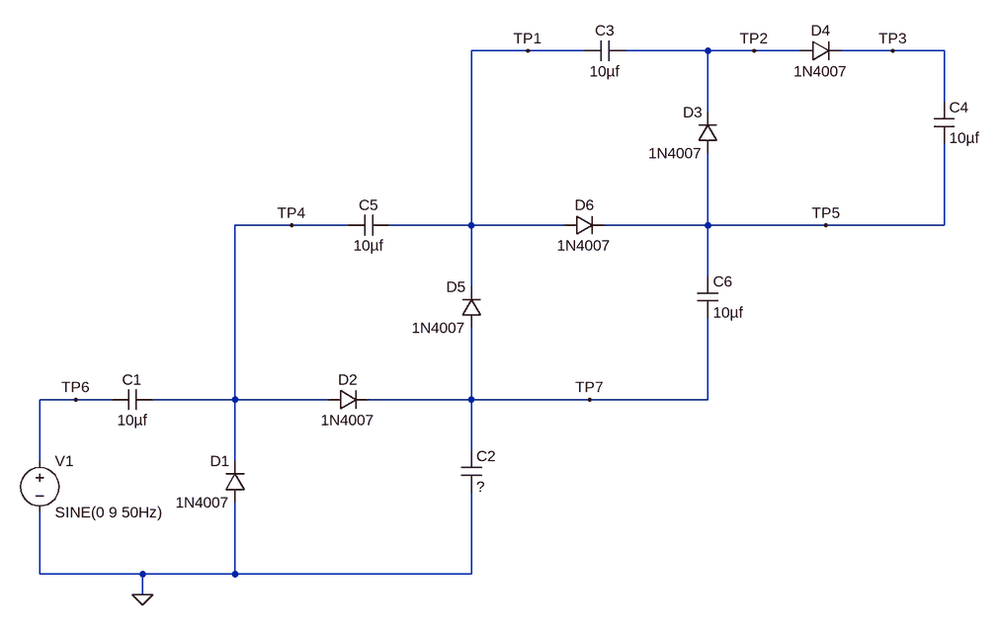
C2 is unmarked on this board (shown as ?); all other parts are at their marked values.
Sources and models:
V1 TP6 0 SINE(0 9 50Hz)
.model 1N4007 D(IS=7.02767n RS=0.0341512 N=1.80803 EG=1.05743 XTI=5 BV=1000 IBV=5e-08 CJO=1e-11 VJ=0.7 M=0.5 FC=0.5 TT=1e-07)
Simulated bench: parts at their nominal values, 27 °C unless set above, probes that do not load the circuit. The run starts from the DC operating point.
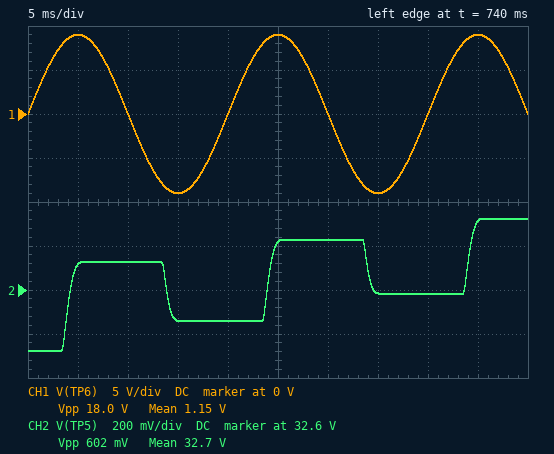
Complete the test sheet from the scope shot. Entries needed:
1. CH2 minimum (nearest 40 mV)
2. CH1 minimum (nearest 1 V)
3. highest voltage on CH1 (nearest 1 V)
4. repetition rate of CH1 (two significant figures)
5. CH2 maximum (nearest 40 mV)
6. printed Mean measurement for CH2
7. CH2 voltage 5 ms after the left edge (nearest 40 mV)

32.32 V
-9 V
9 V
50 Hz
32.92 V
32.7 V
32.72 V
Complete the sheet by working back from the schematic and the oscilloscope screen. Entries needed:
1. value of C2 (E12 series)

33 µF
